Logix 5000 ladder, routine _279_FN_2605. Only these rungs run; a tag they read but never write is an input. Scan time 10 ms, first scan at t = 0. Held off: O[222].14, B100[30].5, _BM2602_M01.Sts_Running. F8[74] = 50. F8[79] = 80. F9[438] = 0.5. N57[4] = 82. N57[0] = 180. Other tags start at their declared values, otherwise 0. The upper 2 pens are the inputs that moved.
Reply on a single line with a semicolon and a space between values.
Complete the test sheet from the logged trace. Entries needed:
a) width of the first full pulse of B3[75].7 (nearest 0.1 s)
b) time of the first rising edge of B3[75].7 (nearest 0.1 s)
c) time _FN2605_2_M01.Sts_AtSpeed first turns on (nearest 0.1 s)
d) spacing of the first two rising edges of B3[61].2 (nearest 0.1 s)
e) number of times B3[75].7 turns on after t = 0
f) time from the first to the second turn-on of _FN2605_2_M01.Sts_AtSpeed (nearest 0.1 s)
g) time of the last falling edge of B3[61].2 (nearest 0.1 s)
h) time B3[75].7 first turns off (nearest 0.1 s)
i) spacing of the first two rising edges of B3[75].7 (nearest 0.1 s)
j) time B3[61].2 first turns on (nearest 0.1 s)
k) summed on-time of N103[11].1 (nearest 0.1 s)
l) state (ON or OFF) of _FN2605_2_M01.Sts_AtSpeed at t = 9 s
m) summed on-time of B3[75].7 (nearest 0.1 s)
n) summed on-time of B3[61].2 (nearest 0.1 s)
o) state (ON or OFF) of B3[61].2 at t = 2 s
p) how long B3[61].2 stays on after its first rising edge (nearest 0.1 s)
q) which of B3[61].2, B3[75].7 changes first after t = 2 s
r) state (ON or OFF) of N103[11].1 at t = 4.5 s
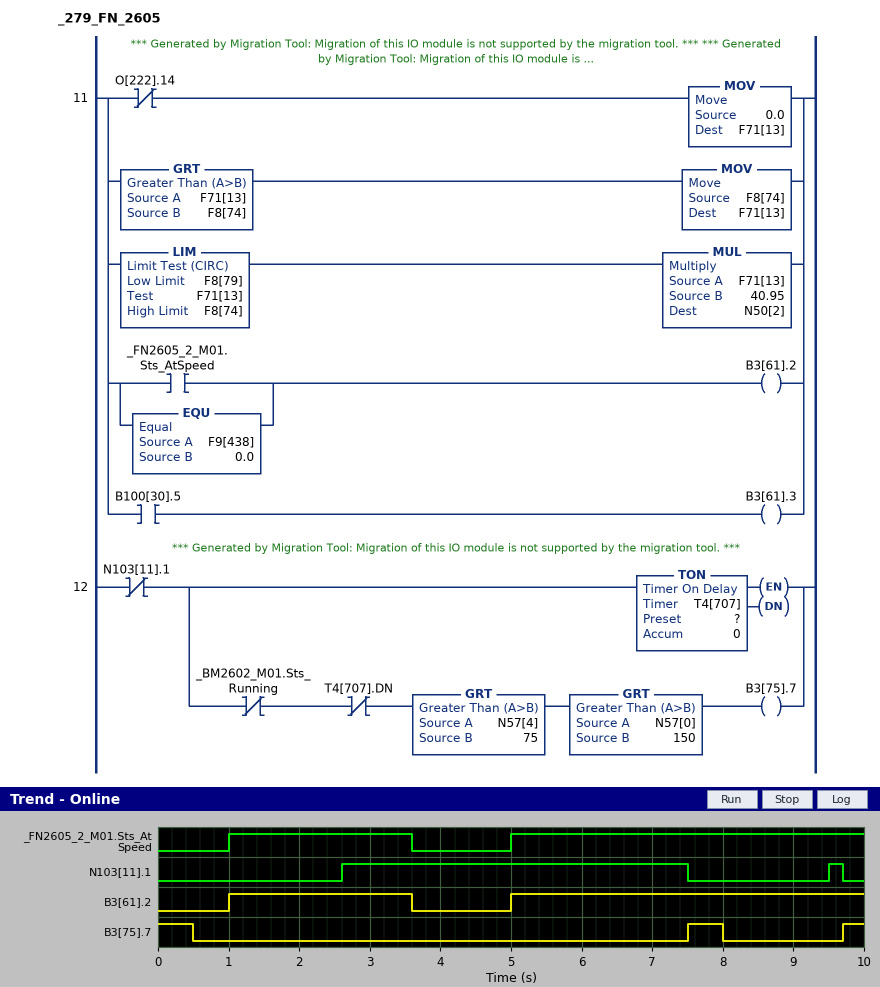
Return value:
0.5 s; 7.5 s; 1.0 s; 4.0 s; 2; 4.0 s; 3.6 s; 0.5 s; 2.2 s; 1.0 s; 5.1 s; ON; 1.3 s; 7.6 s; ON; 2.6 s; B3[61].2; ON
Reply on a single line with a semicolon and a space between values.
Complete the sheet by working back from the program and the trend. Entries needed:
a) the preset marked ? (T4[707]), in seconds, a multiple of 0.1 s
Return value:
0.5 s
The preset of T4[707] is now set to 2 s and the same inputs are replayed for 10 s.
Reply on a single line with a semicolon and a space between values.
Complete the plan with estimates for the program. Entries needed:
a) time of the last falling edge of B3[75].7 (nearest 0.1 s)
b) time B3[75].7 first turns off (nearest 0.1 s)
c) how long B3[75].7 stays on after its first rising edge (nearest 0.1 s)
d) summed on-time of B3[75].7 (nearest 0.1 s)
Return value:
9.5 s; 2.0 s; 2.0 s; 4.3 s
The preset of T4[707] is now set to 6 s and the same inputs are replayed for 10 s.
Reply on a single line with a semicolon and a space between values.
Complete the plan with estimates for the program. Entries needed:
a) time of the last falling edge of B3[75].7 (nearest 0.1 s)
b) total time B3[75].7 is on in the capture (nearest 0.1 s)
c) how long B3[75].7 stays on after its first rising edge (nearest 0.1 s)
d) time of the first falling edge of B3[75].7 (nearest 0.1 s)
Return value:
9.5 s; 4.9 s; 2.0 s; 2.6 s
